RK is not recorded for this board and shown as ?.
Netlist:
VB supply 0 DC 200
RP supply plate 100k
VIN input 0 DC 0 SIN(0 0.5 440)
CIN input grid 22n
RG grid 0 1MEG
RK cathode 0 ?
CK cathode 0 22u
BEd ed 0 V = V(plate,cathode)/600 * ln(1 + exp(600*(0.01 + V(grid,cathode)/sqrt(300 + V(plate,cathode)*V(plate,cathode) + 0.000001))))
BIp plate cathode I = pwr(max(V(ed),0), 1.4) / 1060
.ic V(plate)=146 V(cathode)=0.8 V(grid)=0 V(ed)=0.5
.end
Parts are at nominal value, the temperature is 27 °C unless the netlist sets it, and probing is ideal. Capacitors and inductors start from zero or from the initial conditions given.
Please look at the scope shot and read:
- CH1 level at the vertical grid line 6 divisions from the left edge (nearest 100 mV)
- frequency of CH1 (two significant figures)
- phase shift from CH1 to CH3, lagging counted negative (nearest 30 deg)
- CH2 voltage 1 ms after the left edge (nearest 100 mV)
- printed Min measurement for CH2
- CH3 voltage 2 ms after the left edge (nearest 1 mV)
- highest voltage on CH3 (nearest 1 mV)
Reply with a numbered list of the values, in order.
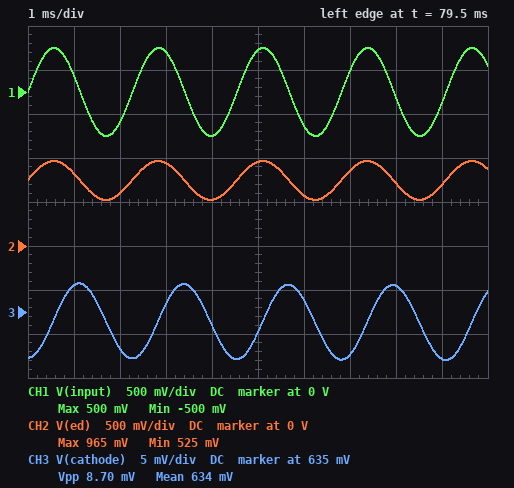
1. -400 mV
2. 440 Hz
3. -90 deg
4. 800 mV
5. 525 mV
6. 631 mV
7. 638 mV
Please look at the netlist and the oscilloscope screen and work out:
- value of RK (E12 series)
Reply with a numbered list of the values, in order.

1. 1 kΩ
